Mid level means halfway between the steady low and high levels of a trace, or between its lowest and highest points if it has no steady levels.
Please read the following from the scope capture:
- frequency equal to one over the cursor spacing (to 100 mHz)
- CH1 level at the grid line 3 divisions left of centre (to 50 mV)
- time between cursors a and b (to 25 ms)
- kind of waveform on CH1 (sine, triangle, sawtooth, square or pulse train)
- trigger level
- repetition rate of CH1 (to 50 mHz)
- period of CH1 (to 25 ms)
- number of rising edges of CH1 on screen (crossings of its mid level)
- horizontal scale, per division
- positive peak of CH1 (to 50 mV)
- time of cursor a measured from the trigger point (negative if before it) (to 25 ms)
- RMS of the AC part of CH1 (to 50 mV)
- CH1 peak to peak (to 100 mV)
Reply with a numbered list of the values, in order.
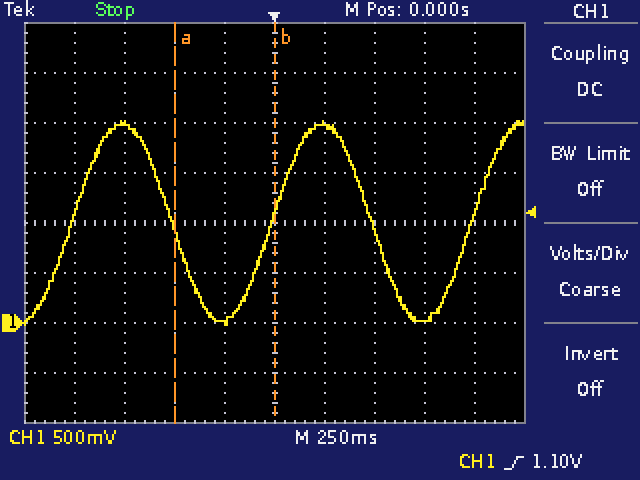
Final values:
1. 2.0 Hz
2. 2.00 V
3. 500 ms
4. sine
5. 1.10 V
6. 1.00 Hz
7. 1.000 s
8. 3
9. 250 ms
10. 2.00 V
11. -500 ms
12. 700 mV
13. 2.00 V
